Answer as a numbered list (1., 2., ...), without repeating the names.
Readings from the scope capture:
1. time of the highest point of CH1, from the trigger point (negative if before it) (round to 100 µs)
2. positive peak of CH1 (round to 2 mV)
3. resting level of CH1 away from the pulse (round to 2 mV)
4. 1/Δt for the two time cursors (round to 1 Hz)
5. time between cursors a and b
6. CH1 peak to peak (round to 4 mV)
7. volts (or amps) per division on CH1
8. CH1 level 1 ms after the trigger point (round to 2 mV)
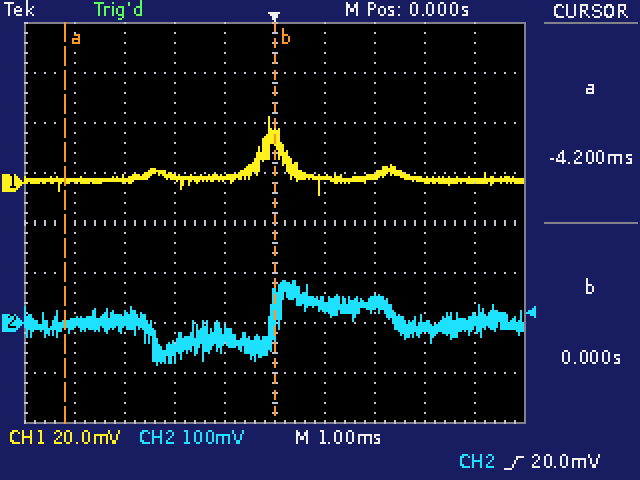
1. -100 µs
2. 26 mV
3. 2 mV
4. 238 Hz
5. 4.2 ms
6. 32 mV
7. 20 mV
8. 2 mV
